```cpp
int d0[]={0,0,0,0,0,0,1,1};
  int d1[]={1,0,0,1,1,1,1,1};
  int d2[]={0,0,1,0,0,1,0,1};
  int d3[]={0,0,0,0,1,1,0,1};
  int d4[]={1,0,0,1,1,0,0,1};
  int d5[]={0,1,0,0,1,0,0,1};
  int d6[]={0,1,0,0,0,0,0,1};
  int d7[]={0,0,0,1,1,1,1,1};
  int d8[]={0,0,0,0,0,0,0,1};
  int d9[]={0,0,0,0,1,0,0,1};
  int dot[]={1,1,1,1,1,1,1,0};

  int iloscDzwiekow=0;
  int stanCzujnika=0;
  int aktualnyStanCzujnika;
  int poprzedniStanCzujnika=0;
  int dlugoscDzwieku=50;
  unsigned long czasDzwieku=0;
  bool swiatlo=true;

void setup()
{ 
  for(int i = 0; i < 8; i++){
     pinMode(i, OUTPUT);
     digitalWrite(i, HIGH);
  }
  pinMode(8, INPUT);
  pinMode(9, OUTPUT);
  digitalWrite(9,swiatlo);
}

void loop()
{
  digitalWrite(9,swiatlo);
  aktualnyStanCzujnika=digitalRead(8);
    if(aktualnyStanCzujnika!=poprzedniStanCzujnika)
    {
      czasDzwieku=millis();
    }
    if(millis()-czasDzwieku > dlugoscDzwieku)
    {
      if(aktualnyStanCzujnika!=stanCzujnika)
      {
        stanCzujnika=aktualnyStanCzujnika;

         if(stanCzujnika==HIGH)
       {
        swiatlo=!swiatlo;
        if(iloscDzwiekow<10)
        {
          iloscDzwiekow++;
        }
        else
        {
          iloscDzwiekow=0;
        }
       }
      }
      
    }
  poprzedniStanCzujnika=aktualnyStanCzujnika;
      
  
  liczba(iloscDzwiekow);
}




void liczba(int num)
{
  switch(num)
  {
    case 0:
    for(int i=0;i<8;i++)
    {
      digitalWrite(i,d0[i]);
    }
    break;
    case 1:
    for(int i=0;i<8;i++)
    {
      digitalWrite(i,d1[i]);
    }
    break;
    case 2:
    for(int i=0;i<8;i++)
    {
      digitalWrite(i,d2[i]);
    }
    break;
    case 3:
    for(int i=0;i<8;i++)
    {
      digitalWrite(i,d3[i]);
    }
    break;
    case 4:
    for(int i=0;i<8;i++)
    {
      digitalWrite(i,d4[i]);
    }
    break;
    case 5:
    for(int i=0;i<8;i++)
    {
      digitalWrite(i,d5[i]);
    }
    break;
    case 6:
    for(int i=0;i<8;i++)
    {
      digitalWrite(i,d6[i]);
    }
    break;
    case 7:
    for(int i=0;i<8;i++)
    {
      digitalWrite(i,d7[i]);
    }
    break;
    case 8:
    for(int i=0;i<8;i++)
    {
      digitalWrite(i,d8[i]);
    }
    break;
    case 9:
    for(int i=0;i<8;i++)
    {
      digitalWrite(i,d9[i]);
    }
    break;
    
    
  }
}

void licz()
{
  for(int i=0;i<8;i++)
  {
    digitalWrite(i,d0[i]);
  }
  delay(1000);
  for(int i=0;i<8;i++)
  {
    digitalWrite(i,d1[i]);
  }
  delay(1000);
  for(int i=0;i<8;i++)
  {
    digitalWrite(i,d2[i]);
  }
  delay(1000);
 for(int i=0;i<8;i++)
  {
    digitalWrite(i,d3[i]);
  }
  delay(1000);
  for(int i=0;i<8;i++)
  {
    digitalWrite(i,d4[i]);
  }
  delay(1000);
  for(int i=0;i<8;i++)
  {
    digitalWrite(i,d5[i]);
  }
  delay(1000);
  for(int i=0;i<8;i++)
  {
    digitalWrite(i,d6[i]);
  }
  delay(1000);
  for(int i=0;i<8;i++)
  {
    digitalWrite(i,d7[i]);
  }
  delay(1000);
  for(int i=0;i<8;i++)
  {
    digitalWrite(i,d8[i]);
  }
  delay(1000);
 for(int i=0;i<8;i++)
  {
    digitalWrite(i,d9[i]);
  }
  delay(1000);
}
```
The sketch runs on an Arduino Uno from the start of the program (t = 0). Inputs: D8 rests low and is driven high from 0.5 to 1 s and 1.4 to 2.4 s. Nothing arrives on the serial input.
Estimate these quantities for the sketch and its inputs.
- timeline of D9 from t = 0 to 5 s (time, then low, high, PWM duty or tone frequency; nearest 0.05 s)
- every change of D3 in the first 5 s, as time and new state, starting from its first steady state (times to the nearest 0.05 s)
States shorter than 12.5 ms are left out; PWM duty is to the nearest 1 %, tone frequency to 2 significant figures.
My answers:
0 s high; 0.55 s low; 1.45 s high
0 s low; 0.55 s high; 1.45 s low
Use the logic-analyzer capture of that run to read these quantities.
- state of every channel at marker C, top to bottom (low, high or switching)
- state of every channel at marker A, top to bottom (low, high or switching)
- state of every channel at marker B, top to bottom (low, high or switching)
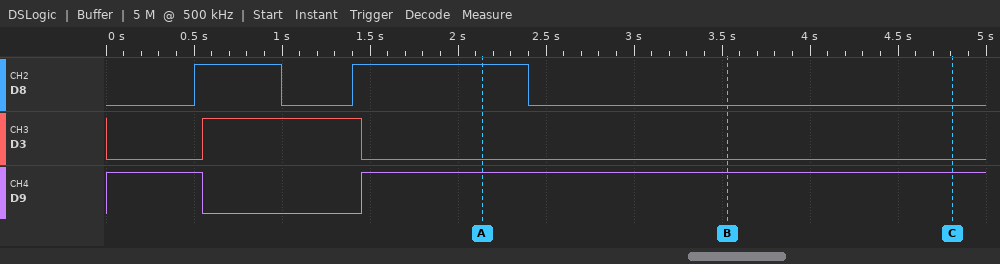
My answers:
D8 low, D3 low, D9 high
D8 high, D3 low, D9 high
D8 low, D3 low, D9 high
